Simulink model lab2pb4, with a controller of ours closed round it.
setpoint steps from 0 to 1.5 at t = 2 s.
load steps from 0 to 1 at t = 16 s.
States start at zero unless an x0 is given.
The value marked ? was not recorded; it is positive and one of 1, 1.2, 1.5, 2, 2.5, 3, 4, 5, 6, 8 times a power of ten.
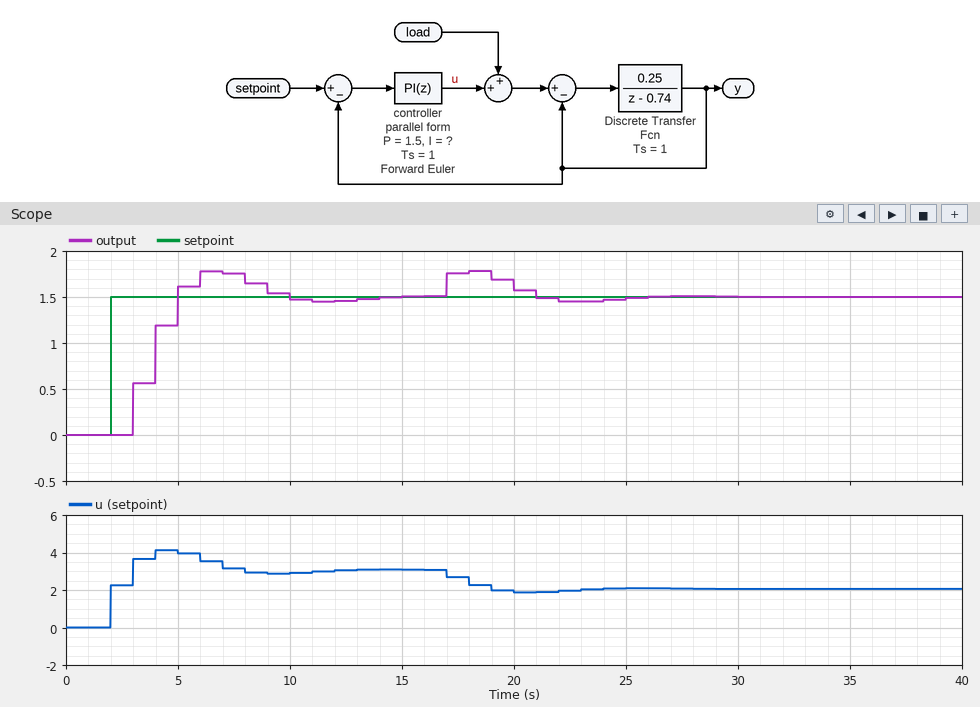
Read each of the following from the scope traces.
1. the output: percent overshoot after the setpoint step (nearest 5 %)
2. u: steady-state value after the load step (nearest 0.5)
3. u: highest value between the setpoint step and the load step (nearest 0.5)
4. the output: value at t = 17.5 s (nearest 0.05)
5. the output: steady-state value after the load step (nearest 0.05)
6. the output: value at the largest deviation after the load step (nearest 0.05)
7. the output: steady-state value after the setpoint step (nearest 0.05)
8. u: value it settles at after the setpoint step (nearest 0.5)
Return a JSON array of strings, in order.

["20 %", "2.0", "4.0", "1.75", "1.50", "1.80", "1.50", "3.0"]
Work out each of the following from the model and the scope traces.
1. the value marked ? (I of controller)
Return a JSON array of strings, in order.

["1.5"]
